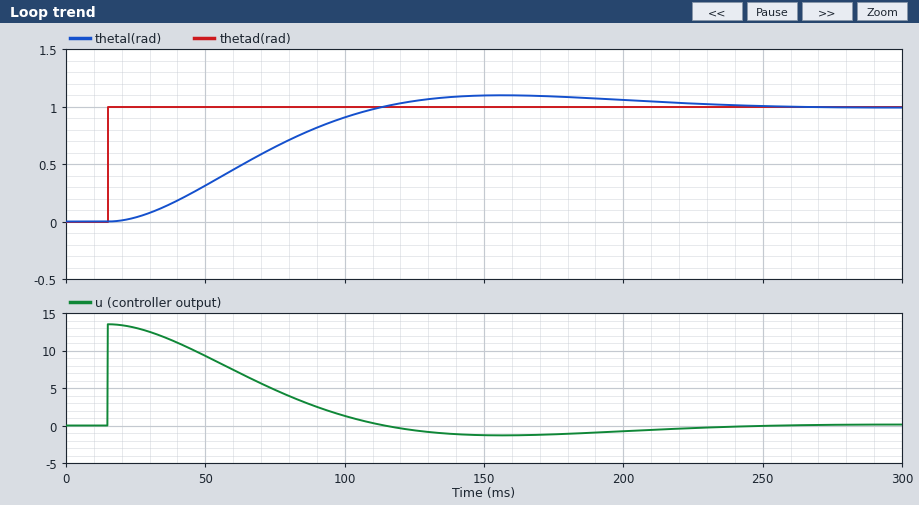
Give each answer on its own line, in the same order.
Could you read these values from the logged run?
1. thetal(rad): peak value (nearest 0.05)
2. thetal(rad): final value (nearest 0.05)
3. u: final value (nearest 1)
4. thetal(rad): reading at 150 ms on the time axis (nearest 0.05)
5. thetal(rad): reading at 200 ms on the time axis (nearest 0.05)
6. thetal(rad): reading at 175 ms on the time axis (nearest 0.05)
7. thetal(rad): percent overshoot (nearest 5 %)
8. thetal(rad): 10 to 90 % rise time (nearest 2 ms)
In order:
1.10
1.00
0
1.10
1.05
1.10
10 %
66 ms
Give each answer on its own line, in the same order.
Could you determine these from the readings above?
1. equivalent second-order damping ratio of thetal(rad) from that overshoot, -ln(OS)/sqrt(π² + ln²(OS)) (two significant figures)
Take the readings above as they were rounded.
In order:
0.59
